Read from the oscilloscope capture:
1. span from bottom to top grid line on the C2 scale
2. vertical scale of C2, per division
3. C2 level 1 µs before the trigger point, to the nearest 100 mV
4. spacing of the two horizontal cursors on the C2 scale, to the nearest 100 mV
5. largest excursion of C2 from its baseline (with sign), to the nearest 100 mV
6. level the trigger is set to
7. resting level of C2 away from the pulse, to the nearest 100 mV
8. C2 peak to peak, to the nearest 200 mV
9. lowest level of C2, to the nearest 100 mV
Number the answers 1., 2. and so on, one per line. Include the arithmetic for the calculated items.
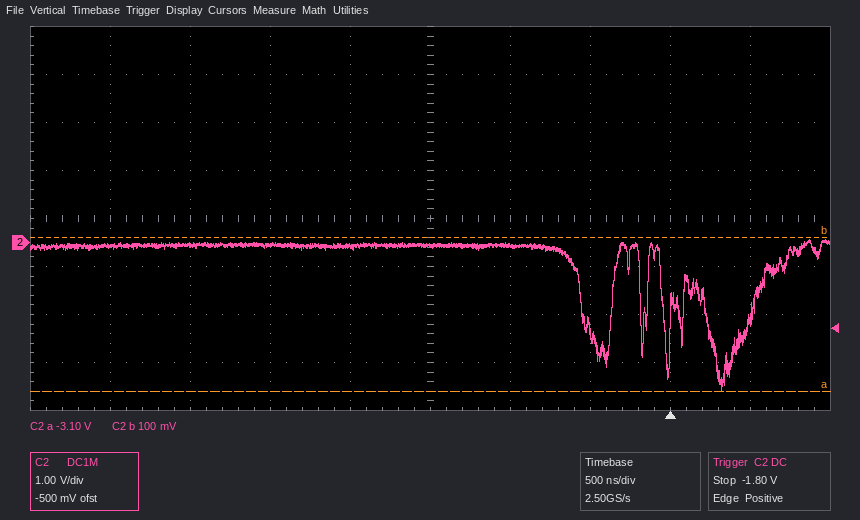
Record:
1. 8 V
2. 1 V
3. -100 mV
4. 3.2 V
5. -3.1 V − (-100 mV) = -3.0 V
6. -1.80 V
7. -100 mV
8. 3.2 V
9. -3.1 V
